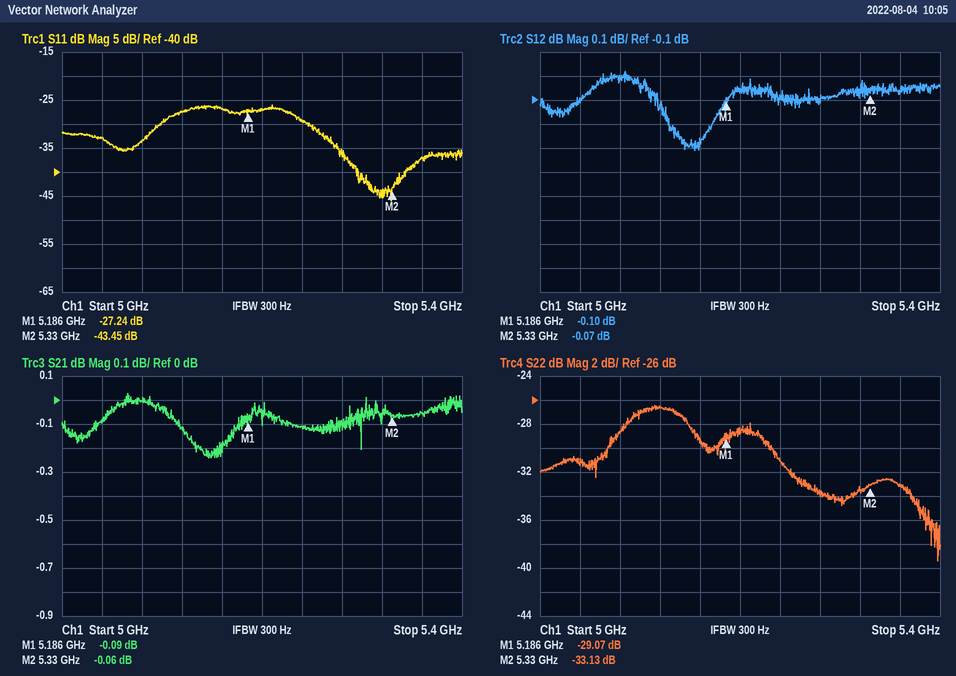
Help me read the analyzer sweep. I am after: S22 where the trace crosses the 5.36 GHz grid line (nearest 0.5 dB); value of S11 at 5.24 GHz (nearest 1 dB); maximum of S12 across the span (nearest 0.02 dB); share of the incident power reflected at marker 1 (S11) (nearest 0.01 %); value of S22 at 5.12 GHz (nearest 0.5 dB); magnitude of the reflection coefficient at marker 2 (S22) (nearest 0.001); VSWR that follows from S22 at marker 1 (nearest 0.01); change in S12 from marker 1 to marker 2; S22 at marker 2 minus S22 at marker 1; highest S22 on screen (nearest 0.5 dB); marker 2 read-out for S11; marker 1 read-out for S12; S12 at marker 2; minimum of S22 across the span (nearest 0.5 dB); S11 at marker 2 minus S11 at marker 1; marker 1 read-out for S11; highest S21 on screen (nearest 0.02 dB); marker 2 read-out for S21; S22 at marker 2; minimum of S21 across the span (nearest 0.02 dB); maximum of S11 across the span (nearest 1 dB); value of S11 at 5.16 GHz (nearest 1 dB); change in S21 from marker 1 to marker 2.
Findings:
-33.0 dB
-29 dB
0.02 dB
0.19 %
-26.5 dB
0.022
1.07
0.03 dB
-4.06 dB
-26.5 dB
-43.45 dB
-0.10 dB
-0.07 dB
-39.5 dB
-16.21 dB
-27.24 dB
0.02 dB
-0.06 dB
-33.13 dB
-0.24 dB
-26 dB
-27 dB
0.03 dB
